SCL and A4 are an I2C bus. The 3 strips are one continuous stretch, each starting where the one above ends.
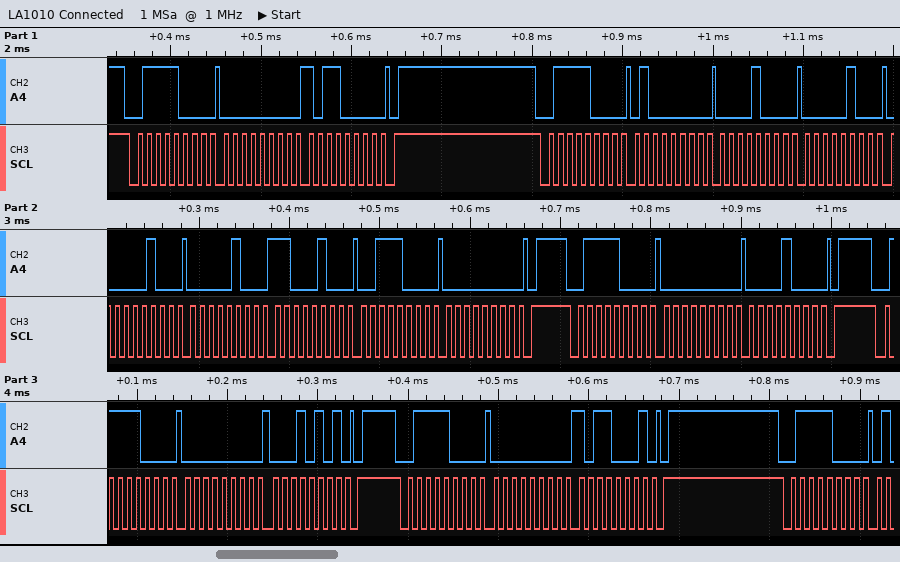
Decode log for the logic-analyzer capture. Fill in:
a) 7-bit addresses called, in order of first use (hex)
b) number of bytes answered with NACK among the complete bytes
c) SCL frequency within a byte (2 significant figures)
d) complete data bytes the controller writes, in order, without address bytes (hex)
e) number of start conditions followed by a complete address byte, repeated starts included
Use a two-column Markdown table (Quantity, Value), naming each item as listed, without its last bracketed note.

| Quantity | Value |
|---|---|
| 7-bit addresses called, in order of first use | 0x3C |
| number of bytes answered with NACK among the complete bytes | 0 |
| SCL frequency within a byte | 100 kHz |
| complete data bytes the controller writes, in order, without address bytes | 00 B0 40 08 04 04 04 C4 38 00 00 08 00 15 00 B1 |
| number of start conditions followed by a complete address byte, repeated starts included | 6 |
